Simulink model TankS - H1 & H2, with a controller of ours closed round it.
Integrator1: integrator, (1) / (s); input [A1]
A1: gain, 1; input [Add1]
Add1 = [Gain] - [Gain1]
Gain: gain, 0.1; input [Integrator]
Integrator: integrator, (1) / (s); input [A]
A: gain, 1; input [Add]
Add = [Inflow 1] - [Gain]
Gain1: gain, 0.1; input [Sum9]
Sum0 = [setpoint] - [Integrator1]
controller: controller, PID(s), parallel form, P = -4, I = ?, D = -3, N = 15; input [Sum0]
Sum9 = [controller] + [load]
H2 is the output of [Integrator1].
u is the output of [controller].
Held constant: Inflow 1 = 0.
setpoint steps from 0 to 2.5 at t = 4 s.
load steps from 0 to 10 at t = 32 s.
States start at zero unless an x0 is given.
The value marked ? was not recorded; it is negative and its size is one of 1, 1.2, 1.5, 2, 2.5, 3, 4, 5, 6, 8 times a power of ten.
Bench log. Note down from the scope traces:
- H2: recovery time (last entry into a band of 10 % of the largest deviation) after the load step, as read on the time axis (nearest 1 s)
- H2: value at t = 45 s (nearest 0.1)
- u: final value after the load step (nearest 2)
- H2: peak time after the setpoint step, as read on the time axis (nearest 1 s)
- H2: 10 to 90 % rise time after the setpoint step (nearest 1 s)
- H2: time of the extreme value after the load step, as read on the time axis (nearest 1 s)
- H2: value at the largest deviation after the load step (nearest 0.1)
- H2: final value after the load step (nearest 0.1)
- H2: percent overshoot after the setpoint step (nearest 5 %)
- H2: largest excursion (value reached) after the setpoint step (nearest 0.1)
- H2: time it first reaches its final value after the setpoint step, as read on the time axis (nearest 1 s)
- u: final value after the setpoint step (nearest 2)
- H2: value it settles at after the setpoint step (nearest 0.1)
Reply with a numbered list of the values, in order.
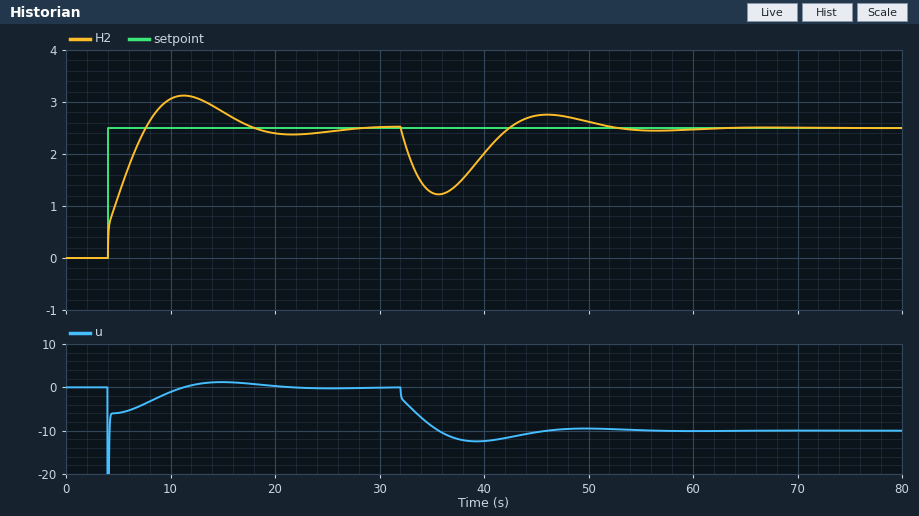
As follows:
1. 50 s
2. 2.7
3. -10
4. 11 s
5. 3 s
6. 36 s
7. 1.2
8. 2.5
9. 25 %
10. 3.1
11. 8 s
12. 0
13. 2.5
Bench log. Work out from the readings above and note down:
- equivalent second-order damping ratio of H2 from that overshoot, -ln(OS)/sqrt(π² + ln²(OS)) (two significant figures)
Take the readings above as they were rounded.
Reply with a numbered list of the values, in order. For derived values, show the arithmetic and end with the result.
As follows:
1. ln(0.25) = -1.386; 1.386 / sqrt(9.870 + 1.922) = 0.40
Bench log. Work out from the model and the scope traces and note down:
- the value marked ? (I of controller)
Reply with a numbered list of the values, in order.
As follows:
1. -1.5
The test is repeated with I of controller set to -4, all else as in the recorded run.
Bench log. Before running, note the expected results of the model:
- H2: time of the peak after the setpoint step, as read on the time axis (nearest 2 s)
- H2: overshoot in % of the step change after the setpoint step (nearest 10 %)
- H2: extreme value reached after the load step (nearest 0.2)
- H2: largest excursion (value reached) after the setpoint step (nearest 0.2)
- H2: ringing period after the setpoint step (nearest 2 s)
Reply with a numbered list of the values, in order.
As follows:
1. 8 s
2. 40 %
3. 1.6
4. 3.4
5. 12 s
